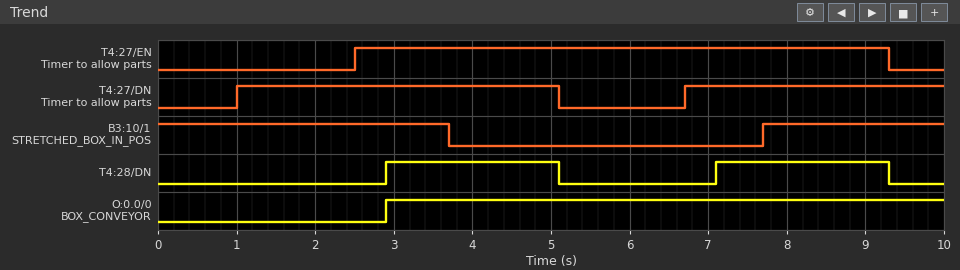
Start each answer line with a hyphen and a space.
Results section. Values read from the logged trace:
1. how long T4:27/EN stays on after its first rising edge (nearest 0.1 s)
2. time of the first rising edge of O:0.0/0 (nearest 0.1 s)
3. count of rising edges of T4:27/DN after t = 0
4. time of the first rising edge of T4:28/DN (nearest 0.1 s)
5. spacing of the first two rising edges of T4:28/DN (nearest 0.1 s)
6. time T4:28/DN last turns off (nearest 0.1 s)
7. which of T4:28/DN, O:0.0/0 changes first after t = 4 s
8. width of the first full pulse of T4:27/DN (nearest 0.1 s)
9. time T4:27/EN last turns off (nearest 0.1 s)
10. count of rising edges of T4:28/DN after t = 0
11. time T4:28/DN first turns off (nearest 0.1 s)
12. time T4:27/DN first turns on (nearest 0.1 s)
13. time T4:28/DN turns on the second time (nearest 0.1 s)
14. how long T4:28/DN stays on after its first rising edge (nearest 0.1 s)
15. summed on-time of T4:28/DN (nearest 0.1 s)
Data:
- 6.8 s
- 2.9 s
- 2
- 2.9 s
- 4.2 s
- 9.3 s
- T4:28/DN
- 4.1 s
- 9.3 s
- 2
- 5.1 s
- 1.0 s
- 7.1 s
- 2.2 s
- 4.4 s
